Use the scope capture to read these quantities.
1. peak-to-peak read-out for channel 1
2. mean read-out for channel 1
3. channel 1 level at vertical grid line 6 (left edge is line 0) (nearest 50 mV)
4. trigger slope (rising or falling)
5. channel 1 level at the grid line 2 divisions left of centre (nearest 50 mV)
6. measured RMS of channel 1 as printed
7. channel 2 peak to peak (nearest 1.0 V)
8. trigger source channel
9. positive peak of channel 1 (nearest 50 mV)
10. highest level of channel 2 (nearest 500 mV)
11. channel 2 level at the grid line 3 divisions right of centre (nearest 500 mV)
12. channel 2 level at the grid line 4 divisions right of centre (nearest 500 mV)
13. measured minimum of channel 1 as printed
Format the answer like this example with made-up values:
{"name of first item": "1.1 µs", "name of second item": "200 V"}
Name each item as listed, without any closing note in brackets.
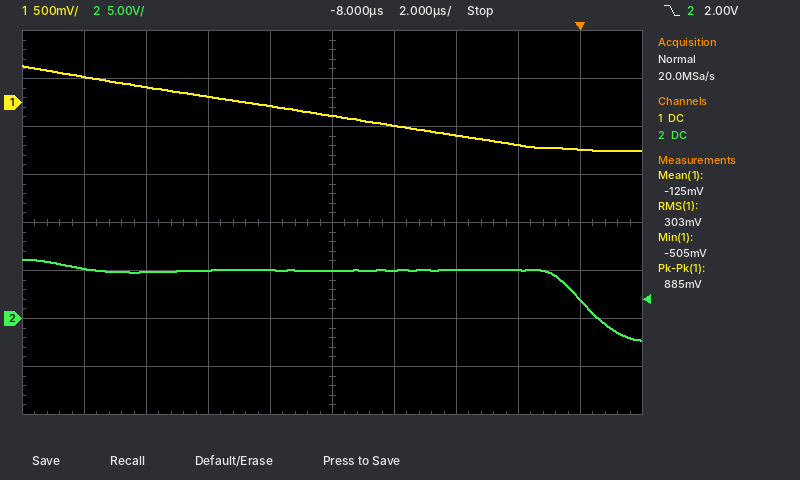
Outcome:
{"peak-to-peak read-out for channel 1": "885 mV", "mean read-out for channel 1": "-125 mV", "channel 1 level at vertical grid line 6 (left edge is line 0)": "-250 mV", "trigger slope": "falling", "channel 1 level at the grid line 2 divisions left of centre": "50 mV", "measured RMS of channel 1 as printed": "303 mV", "channel 2 peak to peak": "8.0 V", "trigger source channel": "channel 2", "positive peak of channel 1": "400 mV", "highest level of channel 2": "6.0 V", "channel 2 level at the grid line 3 divisions right of centre": "5.0 V", "channel 2 level at the grid line 4 divisions right of centre": "2.0 V", "measured minimum of channel 1 as printed": "-505 mV"}
